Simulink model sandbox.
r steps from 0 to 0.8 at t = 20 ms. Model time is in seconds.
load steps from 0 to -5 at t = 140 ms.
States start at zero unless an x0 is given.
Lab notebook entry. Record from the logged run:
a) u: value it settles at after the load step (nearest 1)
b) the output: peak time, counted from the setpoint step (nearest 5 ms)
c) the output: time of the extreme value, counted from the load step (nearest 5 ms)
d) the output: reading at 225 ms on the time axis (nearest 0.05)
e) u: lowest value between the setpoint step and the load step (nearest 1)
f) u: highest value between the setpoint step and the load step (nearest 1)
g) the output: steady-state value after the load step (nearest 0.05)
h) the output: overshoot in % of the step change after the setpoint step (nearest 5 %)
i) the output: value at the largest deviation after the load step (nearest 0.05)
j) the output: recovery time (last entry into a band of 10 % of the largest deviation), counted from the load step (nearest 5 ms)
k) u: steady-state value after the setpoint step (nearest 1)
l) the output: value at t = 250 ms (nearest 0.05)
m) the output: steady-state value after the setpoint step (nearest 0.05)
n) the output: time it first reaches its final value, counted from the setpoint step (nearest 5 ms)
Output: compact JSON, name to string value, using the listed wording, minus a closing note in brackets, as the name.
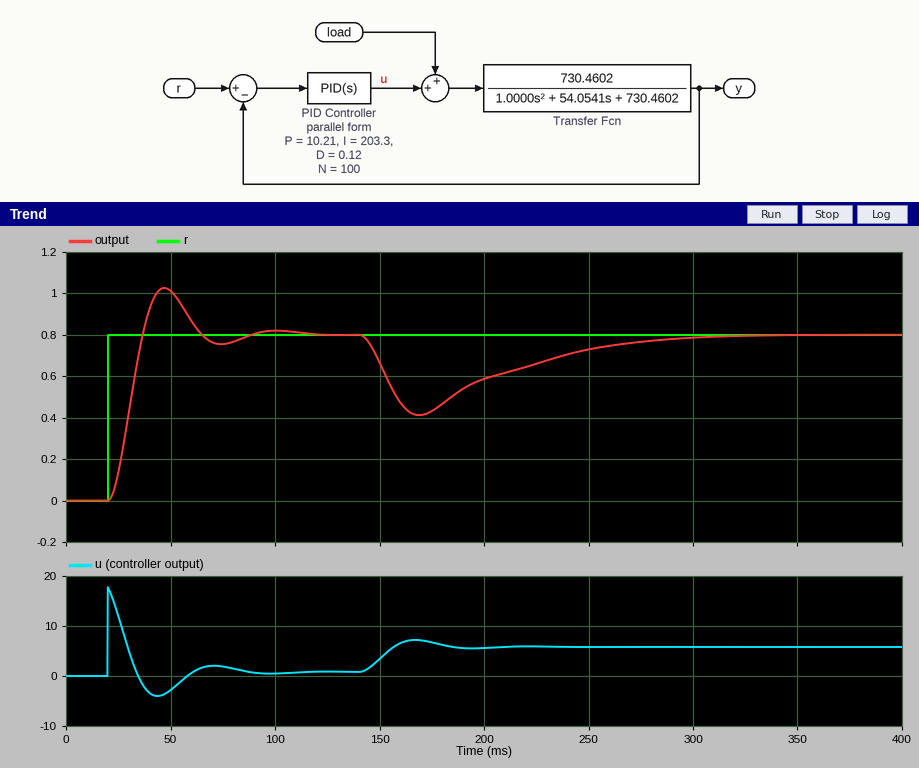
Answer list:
{"u: value it settles at after the load step": "6", "the output: peak time, counted from the setpoint step": "25 ms", "the output: time of the extreme value, counted from the load step": "30 ms", "the output: reading at 225 ms on the time axis": "0.65", "u: lowest value between the setpoint step and the load step": "-4", "u: highest value between the setpoint step and the load step": "18", "the output: steady-state value after the load step": "0.80", "the output: overshoot in % of the step change after the setpoint step": "30 %", "the output: value at the largest deviation after the load step": "0.40", "the output: recovery time (last entry into a band of 10 % of the largest deviation), counted from the load step": "130 ms", "u: steady-state value after the setpoint step": "1", "the output: value at t = 250 ms": "0.75", "the output: steady-state value after the setpoint step": "0.80", "the output: time it first reaches its final value, counted from the setpoint step": "15 ms"}
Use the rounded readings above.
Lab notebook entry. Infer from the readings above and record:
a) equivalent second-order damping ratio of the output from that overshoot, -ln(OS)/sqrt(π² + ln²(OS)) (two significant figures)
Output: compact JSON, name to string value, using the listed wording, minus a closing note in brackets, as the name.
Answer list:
{"equivalent second-order damping ratio of the output from that overshoot, -ln(OS)/sqrt(π² + ln²(OS))": "0.36"}
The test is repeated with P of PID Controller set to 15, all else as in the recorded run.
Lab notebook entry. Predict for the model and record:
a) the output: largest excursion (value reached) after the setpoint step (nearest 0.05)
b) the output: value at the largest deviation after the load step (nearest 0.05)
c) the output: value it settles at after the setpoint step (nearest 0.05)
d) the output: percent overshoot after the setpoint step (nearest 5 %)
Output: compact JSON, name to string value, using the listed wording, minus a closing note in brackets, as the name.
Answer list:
{"the output: largest excursion (value reached) after the setpoint step": "1.10", "the output: value at the largest deviation after the load step": "0.50", "the output: value it settles at after the setpoint step": "0.80", "the output: percent overshoot after the setpoint step": "35 %"}
